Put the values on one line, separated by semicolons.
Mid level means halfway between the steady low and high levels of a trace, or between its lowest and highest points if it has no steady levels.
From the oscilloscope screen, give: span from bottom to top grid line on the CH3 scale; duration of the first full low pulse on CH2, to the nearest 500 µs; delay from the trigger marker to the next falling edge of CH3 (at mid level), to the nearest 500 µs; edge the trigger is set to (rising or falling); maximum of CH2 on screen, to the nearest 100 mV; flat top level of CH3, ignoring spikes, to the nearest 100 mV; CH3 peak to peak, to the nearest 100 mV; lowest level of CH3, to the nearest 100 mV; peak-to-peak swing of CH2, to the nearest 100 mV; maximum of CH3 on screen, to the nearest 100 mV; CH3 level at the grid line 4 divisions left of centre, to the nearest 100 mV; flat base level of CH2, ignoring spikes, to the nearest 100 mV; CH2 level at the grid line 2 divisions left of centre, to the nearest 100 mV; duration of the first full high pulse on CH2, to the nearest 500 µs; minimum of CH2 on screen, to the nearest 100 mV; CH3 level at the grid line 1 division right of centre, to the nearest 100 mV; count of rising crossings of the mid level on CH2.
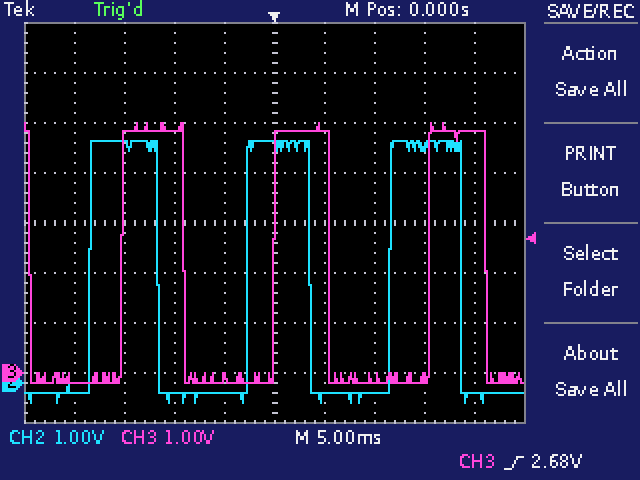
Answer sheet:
8 V; 9.0 ms; 5.5 ms; rising; 4.8 V; 4.8 V; 5.2 V; -200 mV; 5.2 V; 5.0 V; -200 mV; -200 mV; -200 mV; 7.0 ms; -400 mV; 4.8 V; 3
